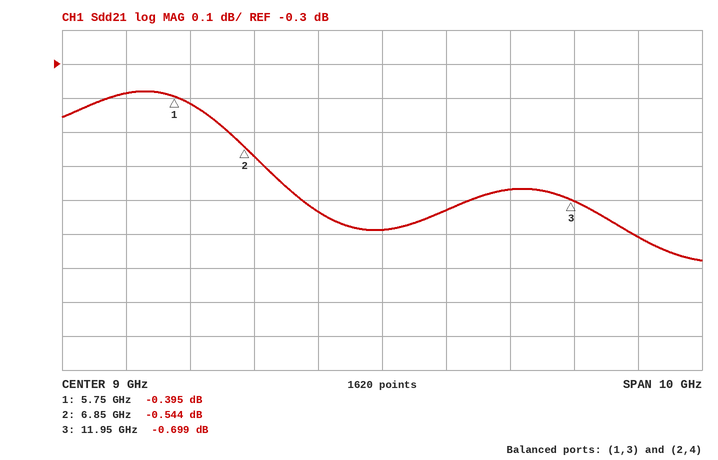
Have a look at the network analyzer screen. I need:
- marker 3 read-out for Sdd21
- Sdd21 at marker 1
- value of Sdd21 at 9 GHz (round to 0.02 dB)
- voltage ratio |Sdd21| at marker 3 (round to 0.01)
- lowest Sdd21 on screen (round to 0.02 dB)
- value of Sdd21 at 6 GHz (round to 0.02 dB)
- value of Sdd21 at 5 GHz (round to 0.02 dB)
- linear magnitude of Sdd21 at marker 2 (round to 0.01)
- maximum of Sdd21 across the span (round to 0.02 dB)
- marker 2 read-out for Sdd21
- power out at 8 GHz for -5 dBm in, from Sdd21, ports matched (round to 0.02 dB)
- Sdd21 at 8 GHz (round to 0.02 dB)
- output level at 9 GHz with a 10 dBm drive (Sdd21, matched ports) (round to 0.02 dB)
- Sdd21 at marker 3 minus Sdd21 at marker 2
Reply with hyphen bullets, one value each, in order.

- -0.699 dB
- -0.395 dB
- -0.78 dB
- 0.92
- -0.88 dB
- -0.42 dB
- -0.38 dB
- 0.94
- -0.38 dB
- -0.544 dB
- -5.74 dBm
- -0.74 dB
- 9.22 dBm
- -0.155 dB
